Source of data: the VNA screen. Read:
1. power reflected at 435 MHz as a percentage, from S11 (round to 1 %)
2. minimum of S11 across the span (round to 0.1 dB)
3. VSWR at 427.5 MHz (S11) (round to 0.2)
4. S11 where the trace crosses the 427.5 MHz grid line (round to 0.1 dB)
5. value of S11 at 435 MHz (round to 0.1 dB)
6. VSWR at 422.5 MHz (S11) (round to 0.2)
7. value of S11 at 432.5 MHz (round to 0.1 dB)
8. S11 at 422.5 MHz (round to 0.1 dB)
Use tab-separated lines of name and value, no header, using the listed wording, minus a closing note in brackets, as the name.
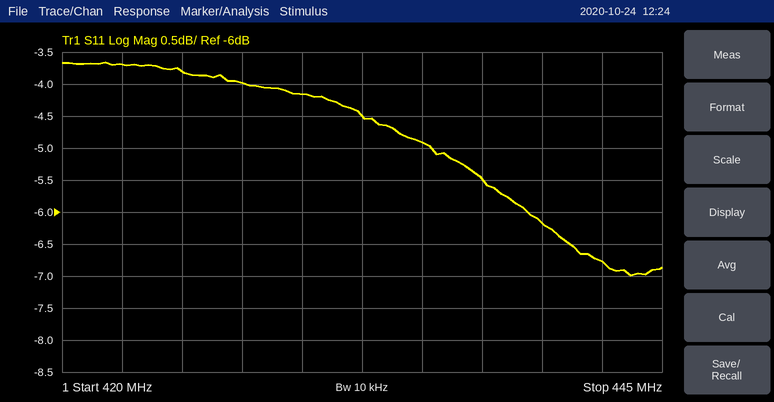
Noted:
power reflected at 435 MHz as a percentage, from S11	32 %
minimum of S11 across the span	-7.0 dB
VSWR at 427.5 MHz (S11)	4.4
S11 where the trace crosses the 427.5 MHz grid line	-4.0 dB
value of S11 at 435 MHz	-4.9 dB
VSWR at 422.5 MHz (S11)	4.8
value of S11 at 432.5 MHz	-4.5 dB
S11 at 422.5 MHz	-3.7 dB
